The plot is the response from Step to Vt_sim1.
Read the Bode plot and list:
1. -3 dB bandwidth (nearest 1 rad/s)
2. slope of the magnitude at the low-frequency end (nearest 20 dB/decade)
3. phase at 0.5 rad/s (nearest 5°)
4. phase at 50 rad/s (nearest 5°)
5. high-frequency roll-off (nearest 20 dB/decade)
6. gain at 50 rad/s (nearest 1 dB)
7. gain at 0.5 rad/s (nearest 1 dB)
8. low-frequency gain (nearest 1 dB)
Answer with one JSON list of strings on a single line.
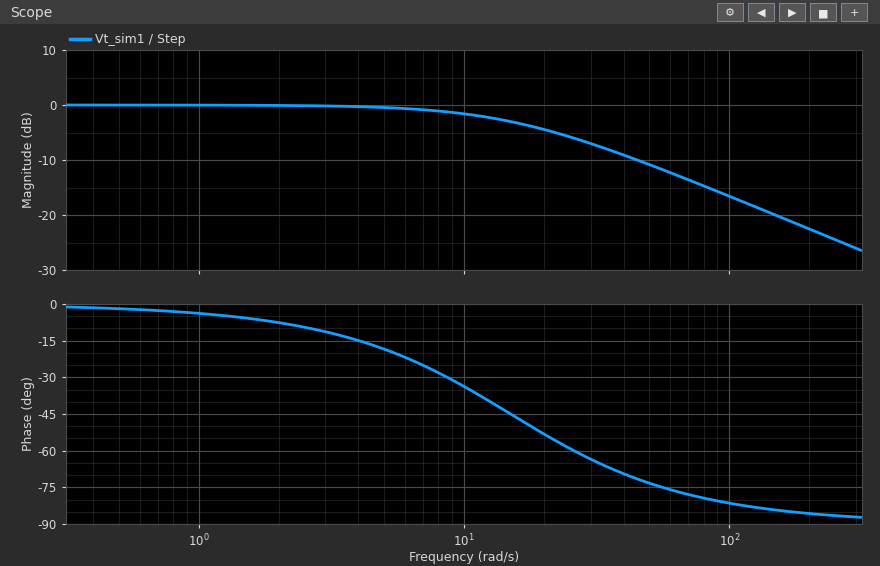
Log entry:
["15 rad/s", "0 dB/decade", "0°", "-75°", "-20 dB/decade", "-11 dB", "0 dB", "0 dB"]
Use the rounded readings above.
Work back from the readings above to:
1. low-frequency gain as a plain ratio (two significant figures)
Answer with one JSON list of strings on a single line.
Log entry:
["1.0"]
